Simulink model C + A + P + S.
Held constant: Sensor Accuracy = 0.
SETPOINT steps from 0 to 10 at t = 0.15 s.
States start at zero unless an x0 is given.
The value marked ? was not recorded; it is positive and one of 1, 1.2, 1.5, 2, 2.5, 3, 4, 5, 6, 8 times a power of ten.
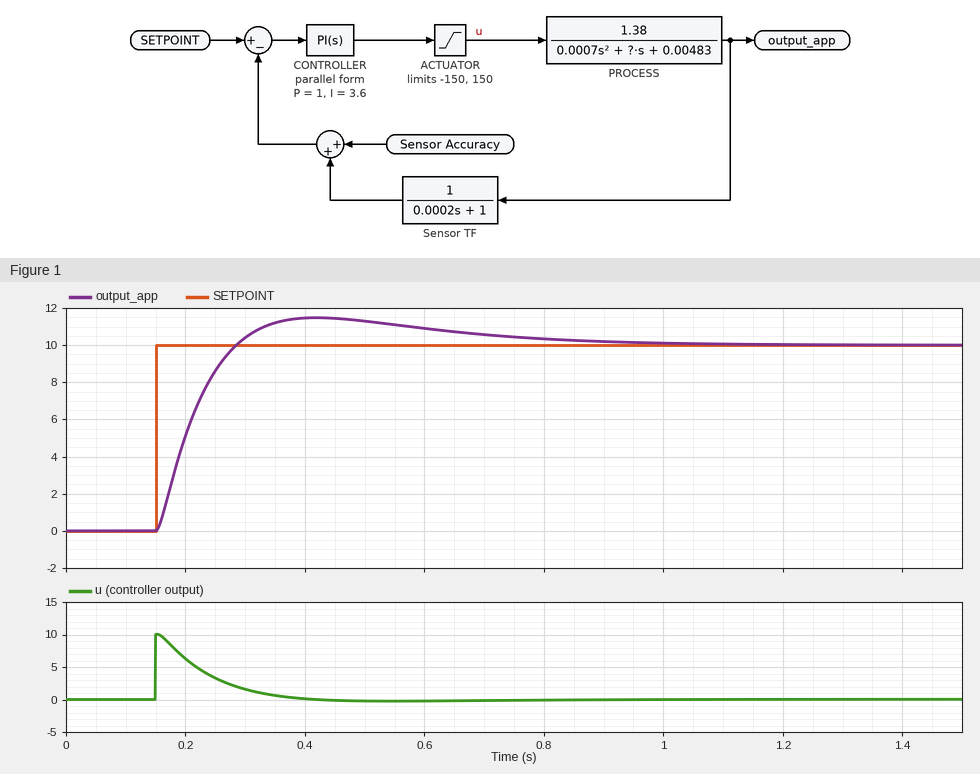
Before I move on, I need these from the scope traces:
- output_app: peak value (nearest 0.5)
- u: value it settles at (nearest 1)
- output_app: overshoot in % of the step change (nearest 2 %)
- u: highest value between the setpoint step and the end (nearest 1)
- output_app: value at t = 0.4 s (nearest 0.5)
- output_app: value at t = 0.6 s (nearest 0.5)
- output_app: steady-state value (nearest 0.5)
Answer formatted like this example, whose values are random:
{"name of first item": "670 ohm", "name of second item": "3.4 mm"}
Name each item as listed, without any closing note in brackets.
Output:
{"output_app: peak value": "11.5", "u: value it settles at": "0", "output_app: overshoot in % of the step change": "14 %", "u: highest value between the setpoint step and the end": "10", "output_app: value at t = 0.4 s": "11.5", "output_app: value at t = 0.6 s": "11.0", "output_app: steady-state value": "10.0"}
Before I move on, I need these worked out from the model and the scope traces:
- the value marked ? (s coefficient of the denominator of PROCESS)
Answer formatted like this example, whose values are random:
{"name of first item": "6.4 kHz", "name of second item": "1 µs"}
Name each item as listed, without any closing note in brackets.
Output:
{"the value marked ?": "0.1"}
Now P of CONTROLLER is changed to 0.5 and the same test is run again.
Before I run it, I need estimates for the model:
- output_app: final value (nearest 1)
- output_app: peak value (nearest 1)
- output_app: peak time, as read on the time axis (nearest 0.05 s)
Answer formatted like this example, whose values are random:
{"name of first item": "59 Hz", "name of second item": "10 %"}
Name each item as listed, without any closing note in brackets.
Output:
{"output_app: final value": "10", "output_app: peak value": "13", "output_app: peak time, as read on the time axis": "0.50 s"}
